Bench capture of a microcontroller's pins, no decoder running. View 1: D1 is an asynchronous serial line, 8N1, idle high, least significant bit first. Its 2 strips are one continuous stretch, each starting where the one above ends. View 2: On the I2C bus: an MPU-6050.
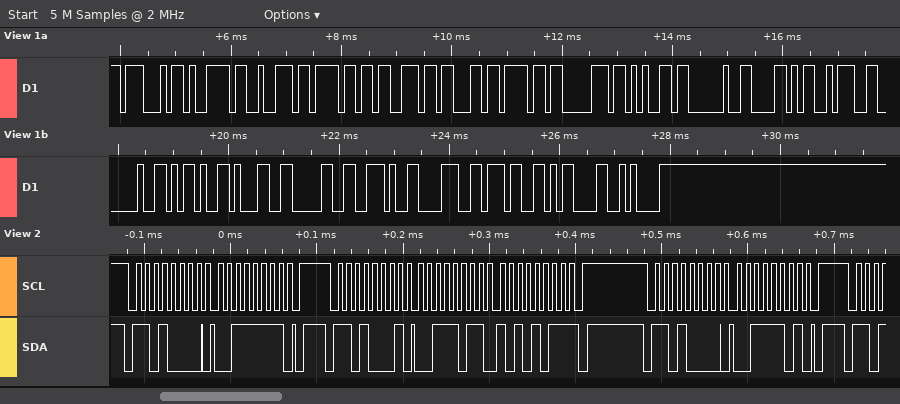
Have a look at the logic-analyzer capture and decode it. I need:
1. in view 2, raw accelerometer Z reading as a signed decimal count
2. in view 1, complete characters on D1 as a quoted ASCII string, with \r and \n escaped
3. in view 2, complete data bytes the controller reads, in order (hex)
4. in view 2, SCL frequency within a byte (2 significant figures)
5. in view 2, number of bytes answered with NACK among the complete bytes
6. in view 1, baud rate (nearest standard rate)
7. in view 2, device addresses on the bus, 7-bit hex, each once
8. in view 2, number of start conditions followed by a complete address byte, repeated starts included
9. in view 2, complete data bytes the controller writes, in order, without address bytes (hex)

15275
"Gyroscope X: -10.87\r\n"
3B AB
100 kHz
1
9600 baud
0x68
3
3F 3D
